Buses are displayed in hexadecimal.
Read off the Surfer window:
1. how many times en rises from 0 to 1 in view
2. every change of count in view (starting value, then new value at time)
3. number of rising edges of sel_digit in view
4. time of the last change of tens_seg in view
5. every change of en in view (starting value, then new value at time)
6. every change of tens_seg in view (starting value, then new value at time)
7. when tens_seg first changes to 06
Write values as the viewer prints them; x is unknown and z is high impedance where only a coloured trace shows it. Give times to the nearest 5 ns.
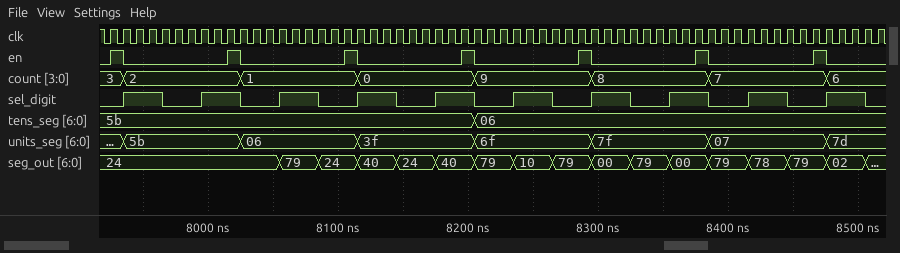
7
3, 2 at 7935 ns, 1 at 8025 ns, 0 at 8115 ns, 9 at 8205 ns, 8 at 8295 ns, 7 at 8385 ns, 6 at 8475 ns
10
8205 ns
0, 1 at 7925 ns, 0 at 7935 ns, 1 at 8015 ns, 0 at 8025 ns, 1 at 8105 ns, 0 at 8115 ns, 1 at 8195 ns, 0 at 8205 ns, 1 at 8285 ns, 0 at 8295 ns, 1 at 8375 ns, 0 at 8385 ns, 1 at 8465 ns, 0 at 8475 ns
5b, 06 at 8205 ns
8205 ns
